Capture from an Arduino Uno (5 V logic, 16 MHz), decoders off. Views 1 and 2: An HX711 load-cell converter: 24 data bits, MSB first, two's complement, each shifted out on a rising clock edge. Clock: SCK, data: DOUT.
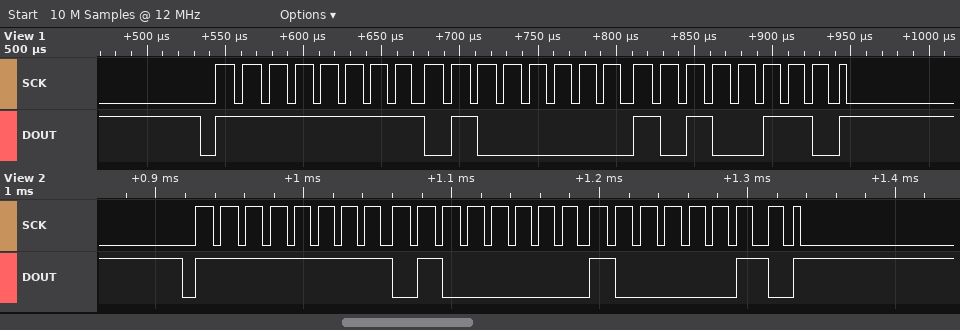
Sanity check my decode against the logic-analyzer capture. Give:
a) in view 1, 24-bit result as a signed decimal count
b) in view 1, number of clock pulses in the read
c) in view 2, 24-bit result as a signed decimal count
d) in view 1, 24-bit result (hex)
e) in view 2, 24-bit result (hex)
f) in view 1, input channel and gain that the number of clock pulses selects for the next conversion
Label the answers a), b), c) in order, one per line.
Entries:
a) -48986
b) 25
c) -49022
d) 0xFF40A6
e) 0xFF4082
f) channel A, gain 128
